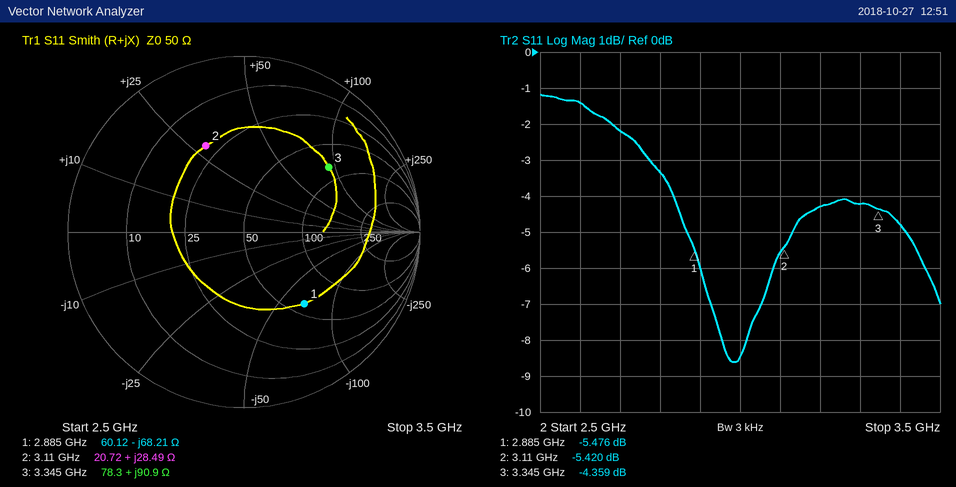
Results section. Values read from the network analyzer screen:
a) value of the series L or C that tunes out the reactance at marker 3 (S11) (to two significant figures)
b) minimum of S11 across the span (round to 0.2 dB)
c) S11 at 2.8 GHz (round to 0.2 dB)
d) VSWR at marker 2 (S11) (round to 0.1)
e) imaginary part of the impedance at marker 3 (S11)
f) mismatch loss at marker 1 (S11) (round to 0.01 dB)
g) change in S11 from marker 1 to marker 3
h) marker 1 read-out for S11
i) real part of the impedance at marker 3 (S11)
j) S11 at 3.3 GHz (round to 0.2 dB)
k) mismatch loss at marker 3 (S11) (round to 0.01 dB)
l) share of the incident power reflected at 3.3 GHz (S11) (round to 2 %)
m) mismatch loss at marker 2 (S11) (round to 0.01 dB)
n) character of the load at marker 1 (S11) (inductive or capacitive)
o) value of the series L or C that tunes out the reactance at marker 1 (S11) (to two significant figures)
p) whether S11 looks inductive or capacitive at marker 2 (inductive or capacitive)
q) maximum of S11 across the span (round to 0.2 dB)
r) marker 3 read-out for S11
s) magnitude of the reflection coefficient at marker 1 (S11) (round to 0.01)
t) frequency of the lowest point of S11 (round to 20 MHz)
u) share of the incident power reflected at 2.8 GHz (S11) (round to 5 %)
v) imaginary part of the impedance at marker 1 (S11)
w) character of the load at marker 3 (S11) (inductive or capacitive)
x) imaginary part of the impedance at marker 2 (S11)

520 fF
-8.6 dB
-3.4 dB
3.3
+90.9 Ω
1.45 dB
1.117 dB
-5.476 dB
78.3 Ω
-4.2 dB
1.98 dB
38 %
1.47 dB
capacitive
3.8 nH
inductive
-1.2 dB
-4.359 dB
0.53
2.98 GHz
45 %
-68.21 Ω
inductive
+28.49 Ω
